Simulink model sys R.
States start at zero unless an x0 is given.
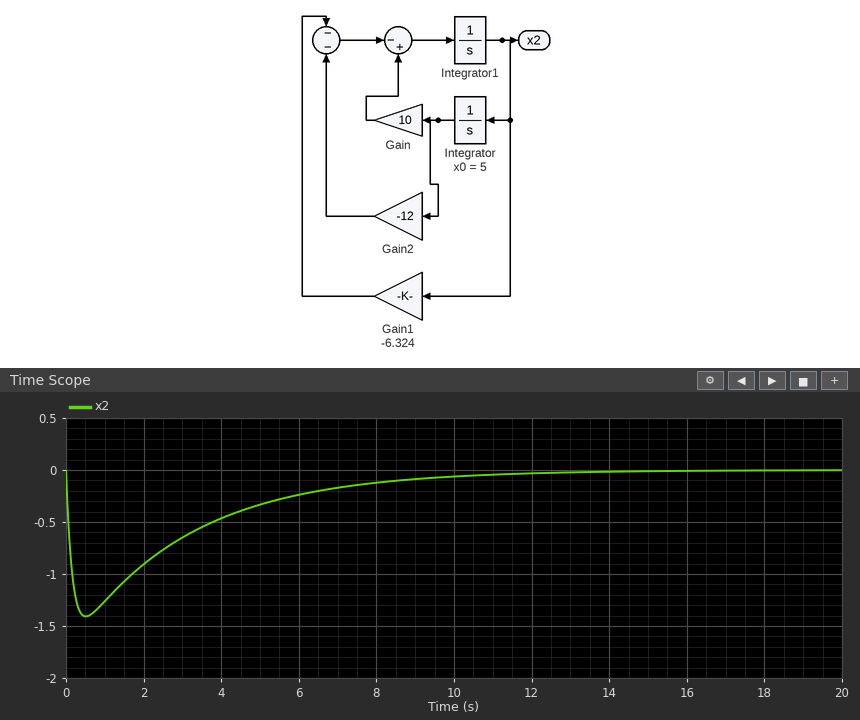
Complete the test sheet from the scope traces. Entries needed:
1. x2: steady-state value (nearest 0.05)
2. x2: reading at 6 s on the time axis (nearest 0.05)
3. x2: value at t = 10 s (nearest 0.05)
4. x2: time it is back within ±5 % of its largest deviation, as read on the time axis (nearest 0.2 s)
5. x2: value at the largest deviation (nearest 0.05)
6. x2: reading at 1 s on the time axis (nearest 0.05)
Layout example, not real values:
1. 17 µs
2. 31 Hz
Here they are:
1. 0.00
2. -0.25
3. -0.05
4. 9.6 s
5. -1.40
6. -1.25
